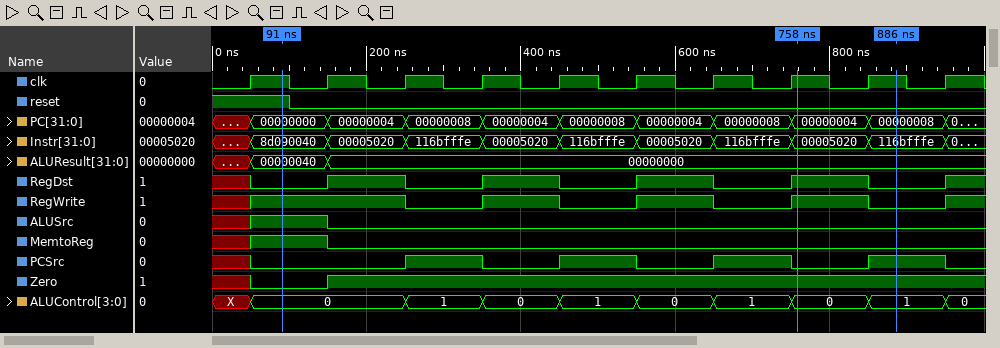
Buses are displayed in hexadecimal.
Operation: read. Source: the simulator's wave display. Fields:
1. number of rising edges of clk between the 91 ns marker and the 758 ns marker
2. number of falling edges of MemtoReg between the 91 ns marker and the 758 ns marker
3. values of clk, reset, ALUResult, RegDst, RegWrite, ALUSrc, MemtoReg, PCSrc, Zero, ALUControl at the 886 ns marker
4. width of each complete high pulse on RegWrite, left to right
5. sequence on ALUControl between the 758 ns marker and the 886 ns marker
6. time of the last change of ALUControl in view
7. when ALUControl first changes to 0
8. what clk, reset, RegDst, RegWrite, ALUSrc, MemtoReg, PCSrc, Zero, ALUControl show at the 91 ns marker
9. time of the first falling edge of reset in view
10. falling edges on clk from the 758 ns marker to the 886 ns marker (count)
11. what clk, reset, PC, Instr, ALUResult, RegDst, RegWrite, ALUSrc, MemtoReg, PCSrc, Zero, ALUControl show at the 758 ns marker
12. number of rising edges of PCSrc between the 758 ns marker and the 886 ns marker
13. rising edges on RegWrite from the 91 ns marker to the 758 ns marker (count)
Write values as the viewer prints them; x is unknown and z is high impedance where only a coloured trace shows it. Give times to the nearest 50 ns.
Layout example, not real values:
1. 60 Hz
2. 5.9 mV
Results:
1. 7
2. 1
3. clk=1, reset=0, ALUResult=00000000, RegDst=0, RegWrite=0, ALUSrc=0, MemtoReg=0, PCSrc=1, Zero=1, ALUControl=1
4. 100 ns, 100 ns, 100 ns
5. 0, 1
6. 950 ns
7. 50 ns
8. clk=1, reset=1, RegDst=0, RegWrite=1, ALUSrc=1, MemtoReg=1, PCSrc=0, Zero=0, ALUControl=0
9. 100 ns
10. 1
11. clk=1, reset=0, PC=00000004, Instr=00005020, ALUResult=00000000, RegDst=1, RegWrite=1, ALUSrc=0, MemtoReg=0, PCSrc=0, Zero=1, ALUControl=0
12. 1
13. 3
